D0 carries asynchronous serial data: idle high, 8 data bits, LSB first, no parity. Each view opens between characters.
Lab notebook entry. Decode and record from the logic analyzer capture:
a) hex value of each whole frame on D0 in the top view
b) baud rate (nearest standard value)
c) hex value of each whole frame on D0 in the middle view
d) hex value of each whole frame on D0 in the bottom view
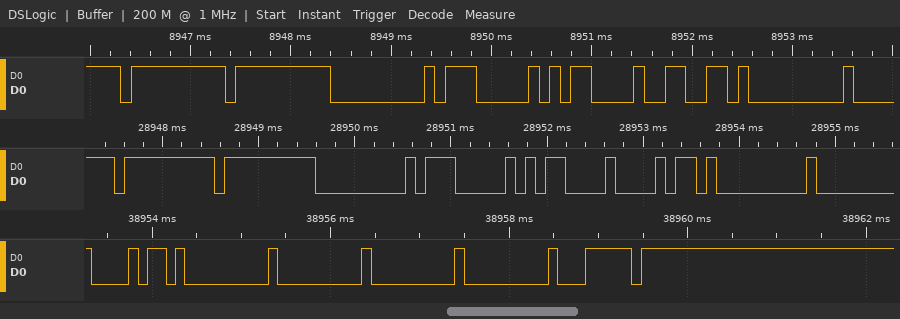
FF, FF, 00, 07, 0D, 66, 00
9600 baud
FF, FF, 00, 07, 0D, 68, 00
68, 00, 00, 00, 00, 7C
